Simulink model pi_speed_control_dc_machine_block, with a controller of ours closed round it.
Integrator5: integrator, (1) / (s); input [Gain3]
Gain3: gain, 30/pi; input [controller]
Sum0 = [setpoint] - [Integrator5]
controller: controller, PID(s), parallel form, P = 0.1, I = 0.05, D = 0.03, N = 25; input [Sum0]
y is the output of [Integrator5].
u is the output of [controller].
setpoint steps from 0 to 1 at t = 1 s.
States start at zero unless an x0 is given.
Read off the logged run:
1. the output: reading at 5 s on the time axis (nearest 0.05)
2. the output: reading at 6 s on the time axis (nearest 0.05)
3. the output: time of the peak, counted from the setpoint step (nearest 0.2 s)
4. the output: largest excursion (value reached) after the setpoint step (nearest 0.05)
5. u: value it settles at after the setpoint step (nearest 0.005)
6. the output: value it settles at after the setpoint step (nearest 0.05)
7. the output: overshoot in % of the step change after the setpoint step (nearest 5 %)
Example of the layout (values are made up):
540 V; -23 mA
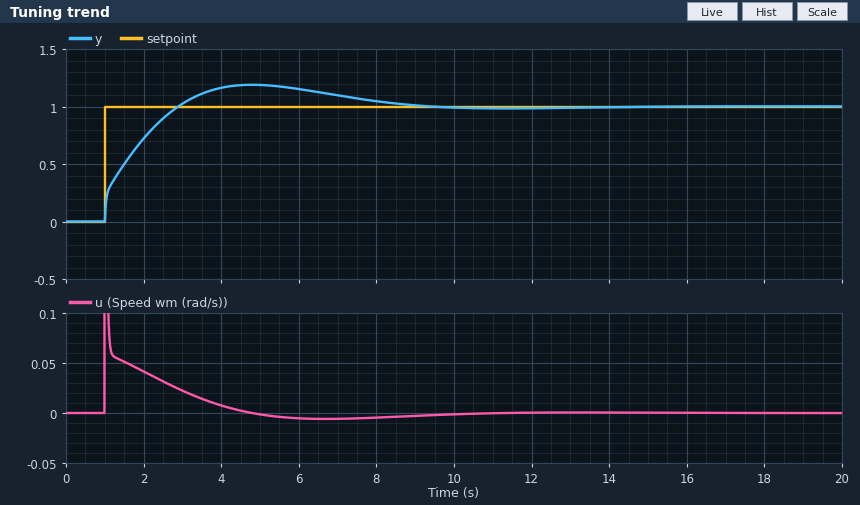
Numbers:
1.20; 1.15; 3.8 s; 1.20; 0.000; 1.00; 20 %
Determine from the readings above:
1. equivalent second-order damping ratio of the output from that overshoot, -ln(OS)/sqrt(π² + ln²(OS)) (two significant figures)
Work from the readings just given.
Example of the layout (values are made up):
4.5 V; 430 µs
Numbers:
0.46
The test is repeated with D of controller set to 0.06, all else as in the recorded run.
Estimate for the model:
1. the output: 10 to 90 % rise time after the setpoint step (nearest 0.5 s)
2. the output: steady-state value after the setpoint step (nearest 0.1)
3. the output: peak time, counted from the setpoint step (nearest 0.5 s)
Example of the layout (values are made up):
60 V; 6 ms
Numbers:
1.5 s; 1.0; 4.5 s
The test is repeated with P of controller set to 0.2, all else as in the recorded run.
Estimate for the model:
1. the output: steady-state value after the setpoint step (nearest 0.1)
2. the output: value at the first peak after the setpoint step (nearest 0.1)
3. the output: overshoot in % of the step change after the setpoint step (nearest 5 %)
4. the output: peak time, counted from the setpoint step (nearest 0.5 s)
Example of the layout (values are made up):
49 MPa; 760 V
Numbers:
1.0; 1.1; 10 %; 3.0 s
